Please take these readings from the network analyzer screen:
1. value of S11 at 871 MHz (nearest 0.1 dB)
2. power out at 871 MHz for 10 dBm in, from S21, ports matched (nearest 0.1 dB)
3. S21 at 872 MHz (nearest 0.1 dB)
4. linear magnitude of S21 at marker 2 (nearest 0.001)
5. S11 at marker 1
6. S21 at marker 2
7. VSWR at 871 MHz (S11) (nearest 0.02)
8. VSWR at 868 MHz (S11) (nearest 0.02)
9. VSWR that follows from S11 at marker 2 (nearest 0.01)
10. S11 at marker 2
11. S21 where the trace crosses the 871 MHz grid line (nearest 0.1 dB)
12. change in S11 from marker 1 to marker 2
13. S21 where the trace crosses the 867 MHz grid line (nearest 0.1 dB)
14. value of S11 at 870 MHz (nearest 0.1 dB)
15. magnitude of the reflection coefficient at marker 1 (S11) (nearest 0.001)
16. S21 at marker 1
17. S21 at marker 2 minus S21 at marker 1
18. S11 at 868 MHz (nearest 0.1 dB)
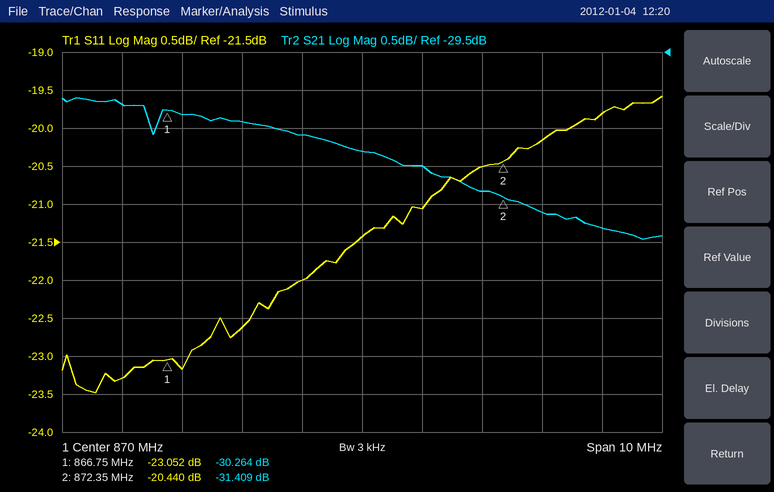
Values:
-21.1 dB
-21.0 dBm
-31.3 dB
0.027
-23.052 dB
-31.409 dB
1.20
1.16
1.21
-20.440 dB
-31.0 dB
2.612 dB
-30.3 dB
-21.4 dB
0.070
-30.264 dB
-1.145 dB
-22.6 dB
